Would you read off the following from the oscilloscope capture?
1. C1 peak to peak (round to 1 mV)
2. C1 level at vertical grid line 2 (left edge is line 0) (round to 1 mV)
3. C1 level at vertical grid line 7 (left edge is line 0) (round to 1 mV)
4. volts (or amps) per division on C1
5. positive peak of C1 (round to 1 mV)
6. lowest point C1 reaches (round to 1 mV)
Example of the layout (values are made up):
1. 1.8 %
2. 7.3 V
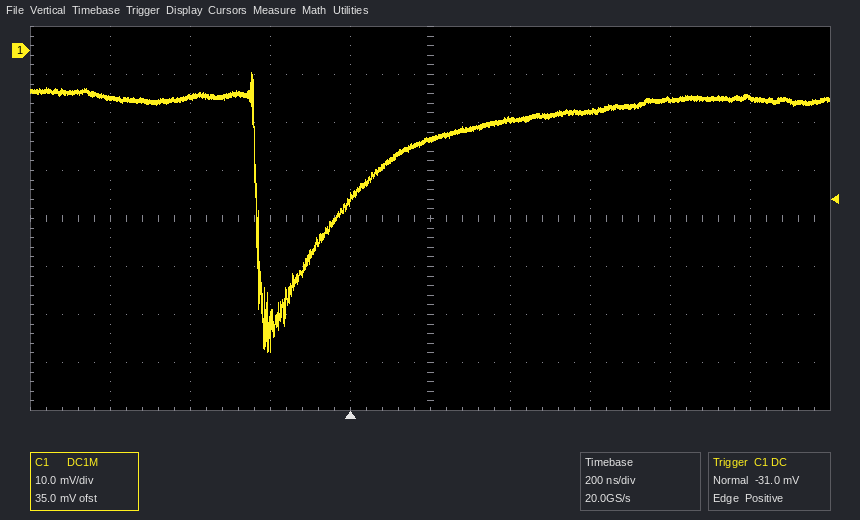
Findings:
1. 58 mV
2. -10 mV
3. -13 mV
4. 10 mV
5. -5 mV
6. -63 mV
